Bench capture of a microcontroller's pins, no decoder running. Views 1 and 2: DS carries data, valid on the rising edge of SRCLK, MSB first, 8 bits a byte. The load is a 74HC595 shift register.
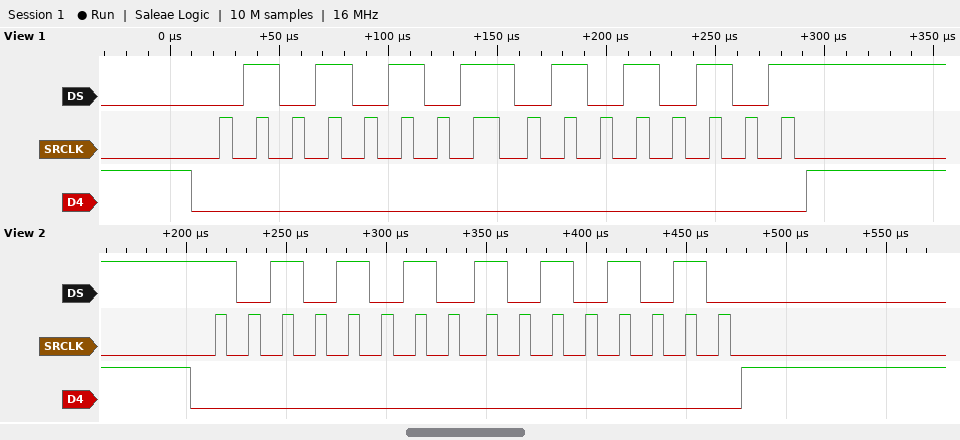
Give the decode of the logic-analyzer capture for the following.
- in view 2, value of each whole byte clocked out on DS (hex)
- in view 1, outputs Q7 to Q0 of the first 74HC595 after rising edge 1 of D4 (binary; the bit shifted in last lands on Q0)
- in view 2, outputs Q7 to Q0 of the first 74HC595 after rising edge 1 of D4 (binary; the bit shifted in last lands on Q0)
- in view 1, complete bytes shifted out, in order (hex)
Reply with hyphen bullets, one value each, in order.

- AA AA
- 01010101
- 10101010
- 55 55
